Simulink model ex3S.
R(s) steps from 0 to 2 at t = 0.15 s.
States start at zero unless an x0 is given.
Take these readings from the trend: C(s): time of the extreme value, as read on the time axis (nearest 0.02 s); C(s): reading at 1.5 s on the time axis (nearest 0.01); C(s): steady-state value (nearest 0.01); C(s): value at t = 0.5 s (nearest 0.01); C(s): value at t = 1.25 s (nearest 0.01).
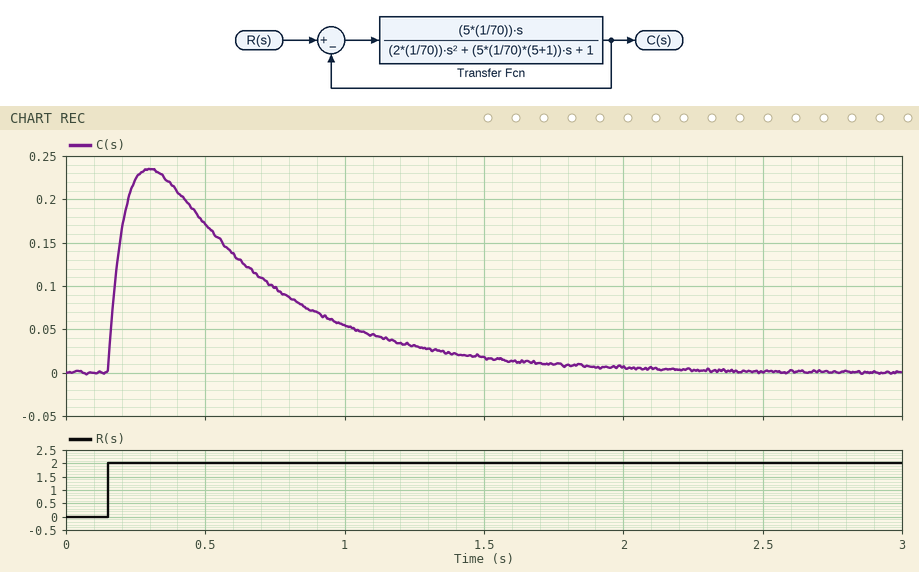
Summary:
0.30 s
0.02
0.00
0.17
0.03
